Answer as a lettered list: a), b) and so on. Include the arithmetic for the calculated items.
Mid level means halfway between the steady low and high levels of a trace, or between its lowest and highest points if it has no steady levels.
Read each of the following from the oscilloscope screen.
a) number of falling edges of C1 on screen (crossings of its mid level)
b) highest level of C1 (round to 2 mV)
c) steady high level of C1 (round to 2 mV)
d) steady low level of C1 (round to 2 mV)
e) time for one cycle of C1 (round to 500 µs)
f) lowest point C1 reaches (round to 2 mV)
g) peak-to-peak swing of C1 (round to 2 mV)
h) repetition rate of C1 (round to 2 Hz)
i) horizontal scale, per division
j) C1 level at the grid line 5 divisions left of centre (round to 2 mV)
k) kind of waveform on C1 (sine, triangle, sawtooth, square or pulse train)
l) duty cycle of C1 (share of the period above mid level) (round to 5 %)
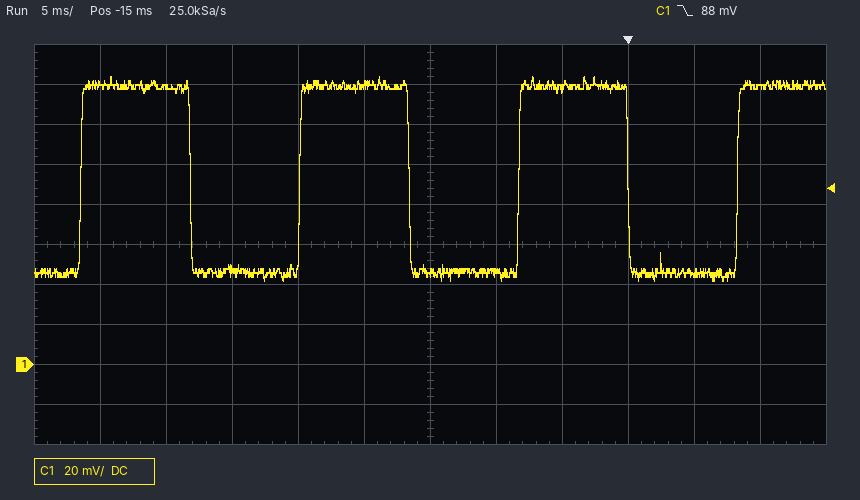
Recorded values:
a) 3
b) 144 mV
c) 140 mV
d) 46 mV
e) 16.5 ms
f) 42 mV
g) 144 mV − (42 mV) = 102 mV
h) 1 / 16.5 ms ≈ 60.6 Hz, so 60 Hz to the nearest 2 Hz
i) 5 ms
j) 140 mV
k) square
l) 50 %
